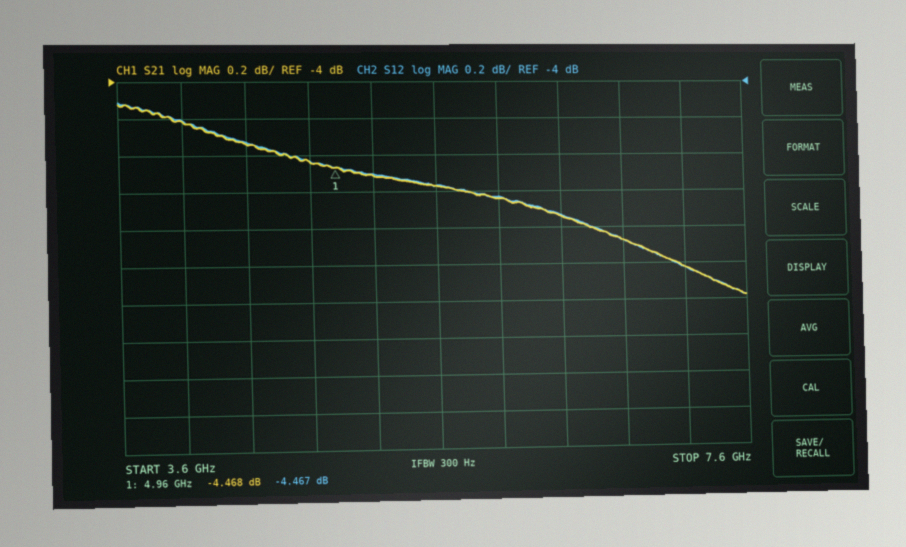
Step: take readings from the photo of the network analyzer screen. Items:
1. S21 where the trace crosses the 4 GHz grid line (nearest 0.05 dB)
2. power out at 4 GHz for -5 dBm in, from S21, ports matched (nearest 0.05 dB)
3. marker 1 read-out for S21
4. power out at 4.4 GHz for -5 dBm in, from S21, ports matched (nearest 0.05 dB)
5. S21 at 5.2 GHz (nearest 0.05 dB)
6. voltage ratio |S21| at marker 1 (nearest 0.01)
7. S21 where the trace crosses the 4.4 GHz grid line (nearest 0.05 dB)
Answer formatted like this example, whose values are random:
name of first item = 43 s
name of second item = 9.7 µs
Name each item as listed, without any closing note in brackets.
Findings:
S21 where the trace crosses the 4 GHz grid line = -4.20 dB
power out at 4 GHz for -5 dBm in, from S21, ports matched = -9.20 dBm
marker 1 read-out for S21 = -4.468 dB
power out at 4.4 GHz for -5 dBm in, from S21, ports matched = -9.35 dBm
S21 at 5.2 GHz = -4.50 dB
voltage ratio |S21| at marker 1 = 0.60
S21 where the trace crosses the 4.4 GHz grid line = -4.35 dB
